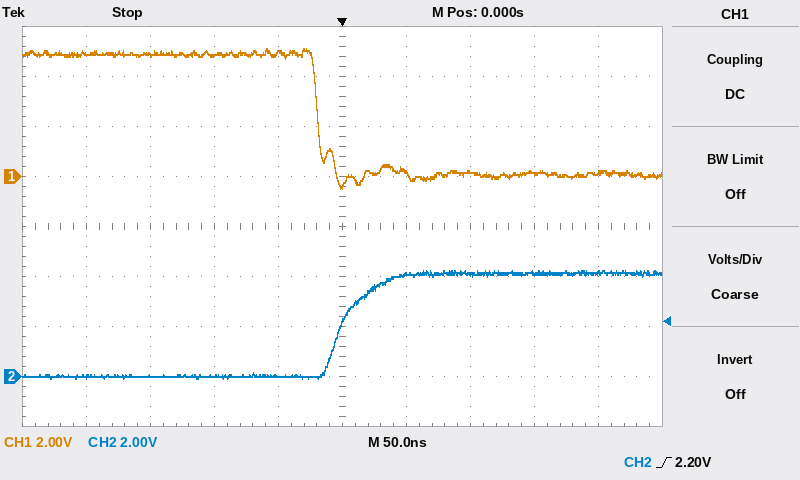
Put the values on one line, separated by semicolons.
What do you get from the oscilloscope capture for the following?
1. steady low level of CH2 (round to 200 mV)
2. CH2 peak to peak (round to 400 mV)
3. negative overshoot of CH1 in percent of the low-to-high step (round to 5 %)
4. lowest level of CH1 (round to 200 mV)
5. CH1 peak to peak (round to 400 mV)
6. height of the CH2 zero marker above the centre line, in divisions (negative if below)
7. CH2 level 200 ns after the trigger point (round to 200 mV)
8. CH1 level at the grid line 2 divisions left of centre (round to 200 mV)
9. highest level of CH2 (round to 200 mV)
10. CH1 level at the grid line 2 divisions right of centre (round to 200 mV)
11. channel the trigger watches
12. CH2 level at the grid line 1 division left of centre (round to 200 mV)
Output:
0.0 V; 4.4 V; 10 %; -400 mV; 5.6 V; -3.0 div; 4.2 V; 4.8 V; 4.2 V; 200 mV; CH2; 0.0 V
